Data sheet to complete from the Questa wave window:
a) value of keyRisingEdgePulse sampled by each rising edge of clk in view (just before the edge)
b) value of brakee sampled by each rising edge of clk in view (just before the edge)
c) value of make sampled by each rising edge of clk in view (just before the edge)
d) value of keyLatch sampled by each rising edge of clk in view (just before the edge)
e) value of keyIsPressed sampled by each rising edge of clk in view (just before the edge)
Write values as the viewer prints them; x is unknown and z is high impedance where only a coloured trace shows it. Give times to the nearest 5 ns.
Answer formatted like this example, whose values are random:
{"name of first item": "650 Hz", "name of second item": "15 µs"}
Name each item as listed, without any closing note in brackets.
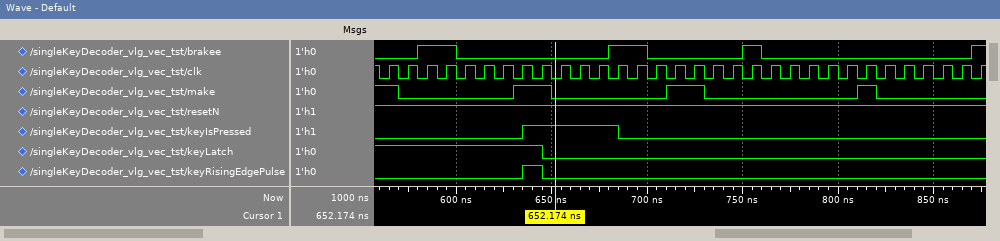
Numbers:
{"value of keyRisingEdgePulse sampled by each rising edge of clk in view": "0 0 0 0 0 0 0 0 1 0 0 0 0 0 0 0 0 0 0 0 0 0 0 0 0 0 0 0 0 0 0 0", "value of brakee sampled by each rising edge of clk in view": "0 0 1 1 0 0 0 0 0 0 0 0 1 1 0 0 0 0 0 1 0 0 0 0 0 0 0 0 0 0 0 1", "value of make sampled by each rising edge of clk in view": "1 0 0 0 0 0 0 1 1 0 0 0 0 0 0 1 1 0 0 0 0 0 0 0 0 1 0 0 0 0 0 0", "value of keyLatch sampled by each rising edge of clk in view": "1 1 1 1 1 1 1 1 1 0 0 0 0 0 0 0 0 0 0 0 0 0 0 0 0 0 0 0 0 0 0 0", "value of keyIsPressed sampled by each rising edge of clk in view": "0 0 0 0 0 0 0 0 1 1 1 1 1 0 0 0 0 0 0 0 0 0 0 0 0 0 0 0 0 0 0 0"}
